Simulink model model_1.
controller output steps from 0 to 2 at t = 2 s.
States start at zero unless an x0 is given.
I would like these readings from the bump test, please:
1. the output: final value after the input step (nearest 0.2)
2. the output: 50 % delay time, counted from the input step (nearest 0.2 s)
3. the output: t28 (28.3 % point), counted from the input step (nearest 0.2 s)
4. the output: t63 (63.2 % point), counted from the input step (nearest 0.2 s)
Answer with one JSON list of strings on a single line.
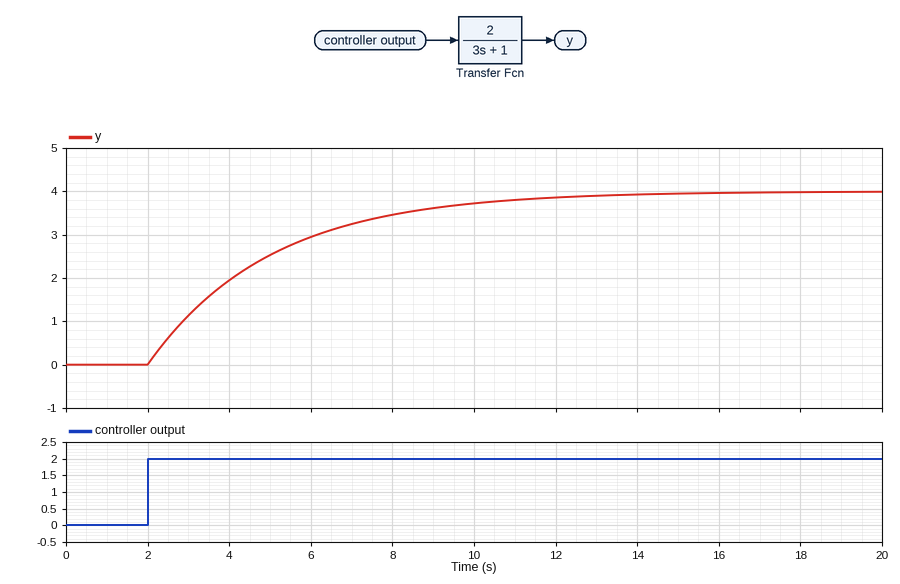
["4.0", "2.0 s", "1.0 s", "3.0 s"]
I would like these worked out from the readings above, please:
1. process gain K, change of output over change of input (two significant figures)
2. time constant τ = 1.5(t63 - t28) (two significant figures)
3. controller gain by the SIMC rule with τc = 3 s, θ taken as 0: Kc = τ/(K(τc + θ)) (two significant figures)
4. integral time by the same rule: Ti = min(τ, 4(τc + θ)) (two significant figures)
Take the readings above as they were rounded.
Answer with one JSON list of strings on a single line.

["2.0", "3.0 s", "0.50", "3.0 s"]
